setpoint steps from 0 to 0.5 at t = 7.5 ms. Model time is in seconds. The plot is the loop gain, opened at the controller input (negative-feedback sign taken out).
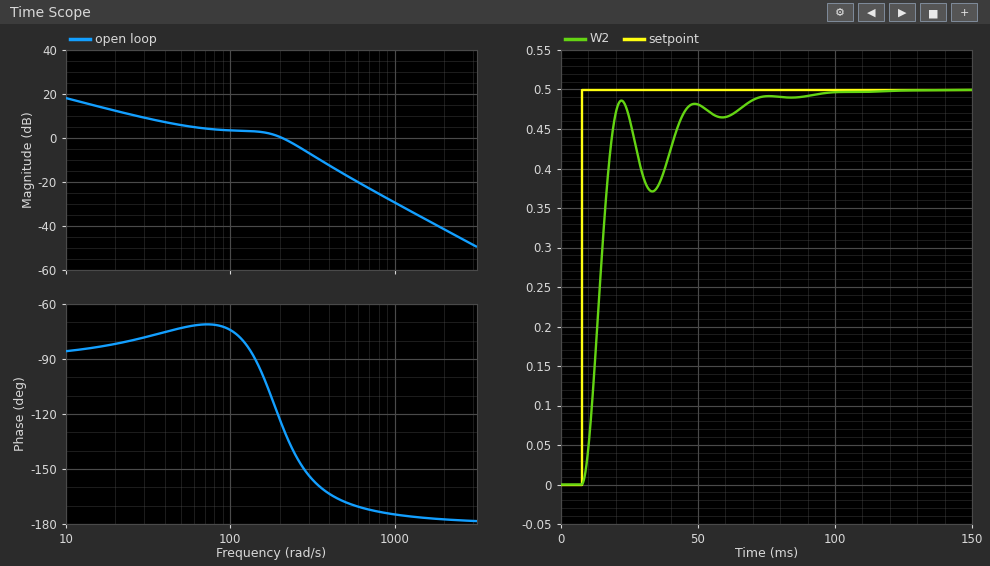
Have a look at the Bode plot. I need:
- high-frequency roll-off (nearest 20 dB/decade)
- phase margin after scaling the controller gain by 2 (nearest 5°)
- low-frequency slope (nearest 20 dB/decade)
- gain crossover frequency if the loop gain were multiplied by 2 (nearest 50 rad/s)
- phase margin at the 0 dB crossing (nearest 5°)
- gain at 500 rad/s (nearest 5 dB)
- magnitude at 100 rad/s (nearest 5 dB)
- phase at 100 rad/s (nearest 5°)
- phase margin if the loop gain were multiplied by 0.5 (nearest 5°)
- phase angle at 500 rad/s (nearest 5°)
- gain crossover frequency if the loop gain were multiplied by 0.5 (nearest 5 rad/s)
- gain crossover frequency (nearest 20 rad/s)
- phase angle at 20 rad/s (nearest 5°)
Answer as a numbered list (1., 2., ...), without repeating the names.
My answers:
1. -40 dB/decade
2. 30°
3. -20 dB/decade
4. 300 rad/s
5. 55°
6. -15 dB
7. 5 dB
8. -75°
9. 105°
10. -170°
11. 50 rad/s
12. 200 rad/s
13. -80°
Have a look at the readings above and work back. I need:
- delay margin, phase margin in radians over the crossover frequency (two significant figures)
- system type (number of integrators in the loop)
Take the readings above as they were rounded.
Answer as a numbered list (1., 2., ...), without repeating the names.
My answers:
1. 0.0048 s
2. 1
